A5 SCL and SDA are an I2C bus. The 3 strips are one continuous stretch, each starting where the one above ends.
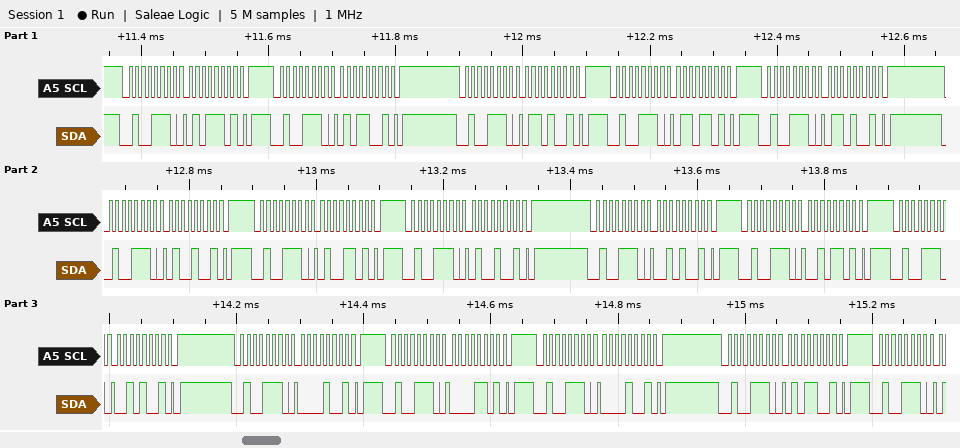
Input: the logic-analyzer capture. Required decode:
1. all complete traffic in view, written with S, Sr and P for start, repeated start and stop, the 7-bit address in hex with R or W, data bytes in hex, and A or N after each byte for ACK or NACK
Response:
S 27W A 5D A P S 27W A 59 A P S 27W A 69 A P S 27W A 6D A P S 27W A 69 A P S 27W A 49 A P S 27W A 4D A P S 27W A 49 A P S 27W A 29 A P S 27W A 2D A P S 27W A 29 A P S 27W A 09 A P S 27W A 0D A P S 27W A 09 A P S 27W A 59 A P S 27W A
